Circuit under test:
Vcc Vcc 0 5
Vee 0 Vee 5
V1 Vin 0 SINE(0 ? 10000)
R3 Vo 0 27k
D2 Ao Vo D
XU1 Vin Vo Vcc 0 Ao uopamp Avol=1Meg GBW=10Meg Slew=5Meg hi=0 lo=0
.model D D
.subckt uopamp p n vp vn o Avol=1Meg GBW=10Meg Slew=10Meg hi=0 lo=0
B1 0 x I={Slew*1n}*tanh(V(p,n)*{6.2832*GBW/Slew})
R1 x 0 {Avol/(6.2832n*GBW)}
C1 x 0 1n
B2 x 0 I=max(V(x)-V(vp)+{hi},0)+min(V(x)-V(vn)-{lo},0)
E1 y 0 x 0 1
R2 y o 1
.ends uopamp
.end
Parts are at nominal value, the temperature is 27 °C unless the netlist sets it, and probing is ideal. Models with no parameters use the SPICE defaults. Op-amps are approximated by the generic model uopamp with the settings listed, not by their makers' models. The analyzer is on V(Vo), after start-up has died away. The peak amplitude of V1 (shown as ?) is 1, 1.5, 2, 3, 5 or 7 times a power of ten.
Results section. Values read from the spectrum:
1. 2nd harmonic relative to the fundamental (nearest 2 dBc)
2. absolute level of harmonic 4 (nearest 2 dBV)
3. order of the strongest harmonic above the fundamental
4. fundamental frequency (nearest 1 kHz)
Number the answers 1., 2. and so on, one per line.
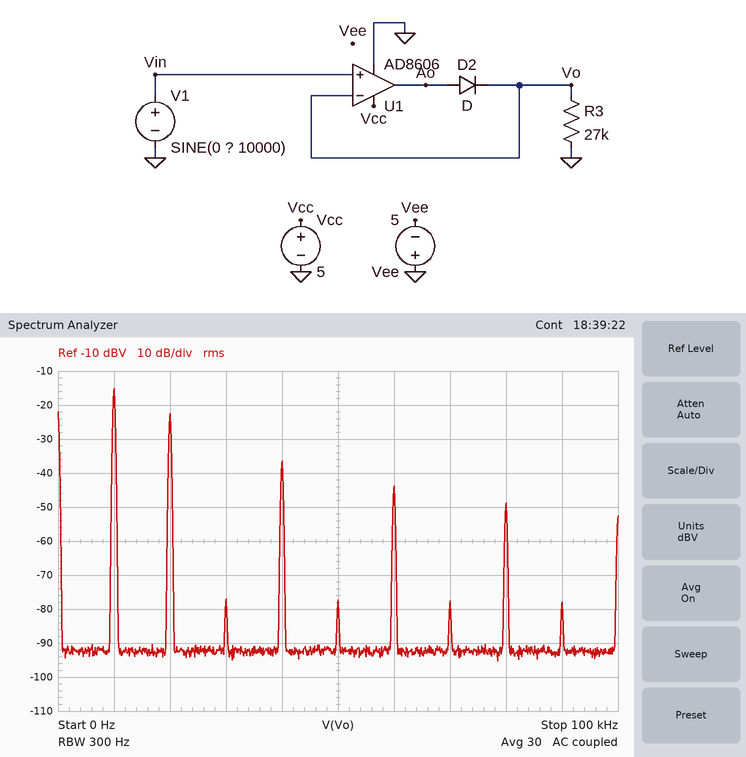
1. -8 dBc
2. -36 dBV
3. 2
4. 10 kHz
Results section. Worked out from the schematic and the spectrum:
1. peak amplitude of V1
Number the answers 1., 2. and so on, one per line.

1. 500 mV
